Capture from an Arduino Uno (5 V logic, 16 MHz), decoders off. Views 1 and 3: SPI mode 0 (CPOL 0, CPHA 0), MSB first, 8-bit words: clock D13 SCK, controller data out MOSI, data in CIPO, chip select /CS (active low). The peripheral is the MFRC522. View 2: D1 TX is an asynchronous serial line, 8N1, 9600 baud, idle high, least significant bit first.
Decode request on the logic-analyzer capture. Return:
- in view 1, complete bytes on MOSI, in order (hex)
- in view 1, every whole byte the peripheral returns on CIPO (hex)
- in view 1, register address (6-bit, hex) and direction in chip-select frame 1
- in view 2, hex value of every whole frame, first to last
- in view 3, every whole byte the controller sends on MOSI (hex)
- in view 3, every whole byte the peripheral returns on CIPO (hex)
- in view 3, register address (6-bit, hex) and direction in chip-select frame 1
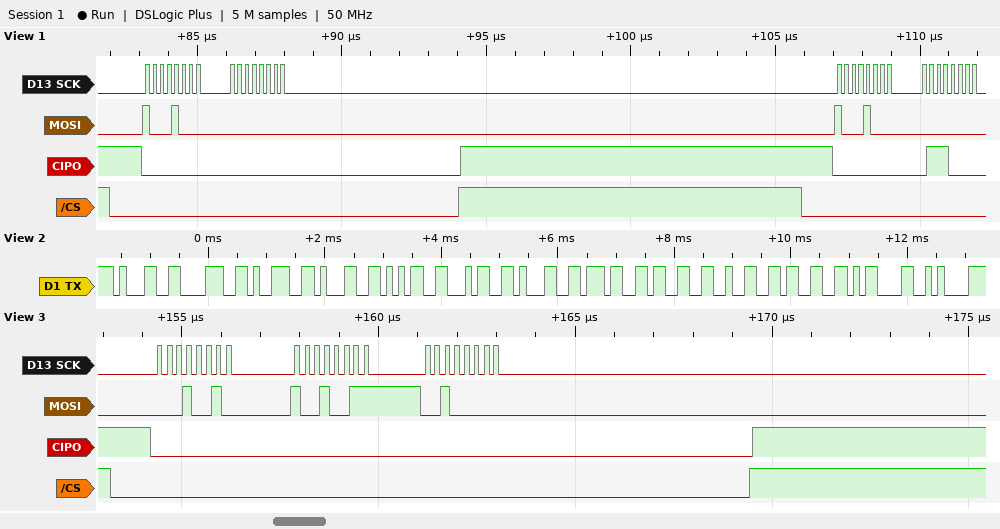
88 00 88 00
00 00 00 70
0x04 read
31 38 39 31 35 34 31 37 33 32 33 0D 0A
0x12 0x93 0x20
0x00 0x00 0x00
0x09 write
